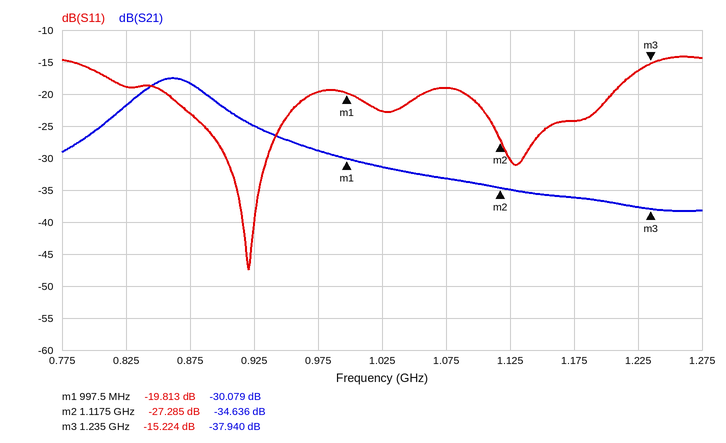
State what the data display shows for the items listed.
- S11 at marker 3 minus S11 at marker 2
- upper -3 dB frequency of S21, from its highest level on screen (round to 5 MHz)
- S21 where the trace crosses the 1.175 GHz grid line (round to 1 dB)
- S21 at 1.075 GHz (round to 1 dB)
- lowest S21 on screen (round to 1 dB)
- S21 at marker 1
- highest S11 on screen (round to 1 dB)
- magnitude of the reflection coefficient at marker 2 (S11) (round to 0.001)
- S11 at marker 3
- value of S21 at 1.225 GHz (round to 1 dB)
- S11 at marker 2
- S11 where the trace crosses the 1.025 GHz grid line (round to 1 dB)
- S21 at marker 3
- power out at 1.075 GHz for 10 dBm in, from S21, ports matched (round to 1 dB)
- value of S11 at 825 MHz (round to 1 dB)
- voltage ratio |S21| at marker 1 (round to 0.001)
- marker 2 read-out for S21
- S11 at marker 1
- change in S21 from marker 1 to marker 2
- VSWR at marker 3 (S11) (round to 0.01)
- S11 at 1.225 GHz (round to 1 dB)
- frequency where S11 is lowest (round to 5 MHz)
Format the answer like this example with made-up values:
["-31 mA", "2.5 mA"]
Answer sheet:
["12.061 dB", "890 MHz", "-36 dB", "-33 dB", "-38 dB", "-30.079 dB", "-14 dB", "0.043", "-15.224 dB", "-38 dB", "-27.285 dB", "-23 dB", "-37.940 dB", "-23 dBm", "-19 dB", "0.031", "-34.636 dB", "-19.813 dB", "-4.557 dB", "1.42", "-16 dB", "920 MHz"]
